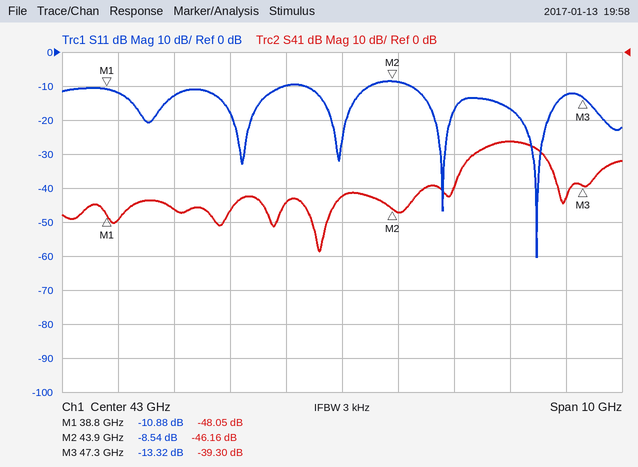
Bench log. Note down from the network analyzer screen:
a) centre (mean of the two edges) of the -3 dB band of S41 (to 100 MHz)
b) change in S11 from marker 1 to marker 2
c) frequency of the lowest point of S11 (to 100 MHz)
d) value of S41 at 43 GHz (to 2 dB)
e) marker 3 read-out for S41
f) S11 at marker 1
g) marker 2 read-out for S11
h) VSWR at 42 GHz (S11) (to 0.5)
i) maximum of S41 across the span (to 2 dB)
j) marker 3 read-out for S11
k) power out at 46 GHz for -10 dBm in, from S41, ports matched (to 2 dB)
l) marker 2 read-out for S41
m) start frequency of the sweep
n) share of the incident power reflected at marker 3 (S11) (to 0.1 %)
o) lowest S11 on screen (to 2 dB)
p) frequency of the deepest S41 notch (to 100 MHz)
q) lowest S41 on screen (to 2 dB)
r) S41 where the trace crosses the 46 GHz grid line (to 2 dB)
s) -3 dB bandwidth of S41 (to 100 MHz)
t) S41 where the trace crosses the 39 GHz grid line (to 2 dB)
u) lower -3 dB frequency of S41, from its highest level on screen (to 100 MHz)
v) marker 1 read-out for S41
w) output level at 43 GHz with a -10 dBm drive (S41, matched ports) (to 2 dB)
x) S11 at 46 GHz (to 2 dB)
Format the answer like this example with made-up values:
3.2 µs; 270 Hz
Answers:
46.0 GHz; 2.34 dB; 46.5 GHz; -42 dB; -39.30 dB; -10.88 dB; -8.54 dB; 2.0; -26 dB; -13.32 dB; -36 dBm; -46.16 dB; 38 GHz; 4.7 %; -60 dB; 42.6 GHz; -58 dB; -26 dB; 1.1 GHz; -50 dB; 45.4 GHz; -48.05 dB; -52 dBm; -16 dB
